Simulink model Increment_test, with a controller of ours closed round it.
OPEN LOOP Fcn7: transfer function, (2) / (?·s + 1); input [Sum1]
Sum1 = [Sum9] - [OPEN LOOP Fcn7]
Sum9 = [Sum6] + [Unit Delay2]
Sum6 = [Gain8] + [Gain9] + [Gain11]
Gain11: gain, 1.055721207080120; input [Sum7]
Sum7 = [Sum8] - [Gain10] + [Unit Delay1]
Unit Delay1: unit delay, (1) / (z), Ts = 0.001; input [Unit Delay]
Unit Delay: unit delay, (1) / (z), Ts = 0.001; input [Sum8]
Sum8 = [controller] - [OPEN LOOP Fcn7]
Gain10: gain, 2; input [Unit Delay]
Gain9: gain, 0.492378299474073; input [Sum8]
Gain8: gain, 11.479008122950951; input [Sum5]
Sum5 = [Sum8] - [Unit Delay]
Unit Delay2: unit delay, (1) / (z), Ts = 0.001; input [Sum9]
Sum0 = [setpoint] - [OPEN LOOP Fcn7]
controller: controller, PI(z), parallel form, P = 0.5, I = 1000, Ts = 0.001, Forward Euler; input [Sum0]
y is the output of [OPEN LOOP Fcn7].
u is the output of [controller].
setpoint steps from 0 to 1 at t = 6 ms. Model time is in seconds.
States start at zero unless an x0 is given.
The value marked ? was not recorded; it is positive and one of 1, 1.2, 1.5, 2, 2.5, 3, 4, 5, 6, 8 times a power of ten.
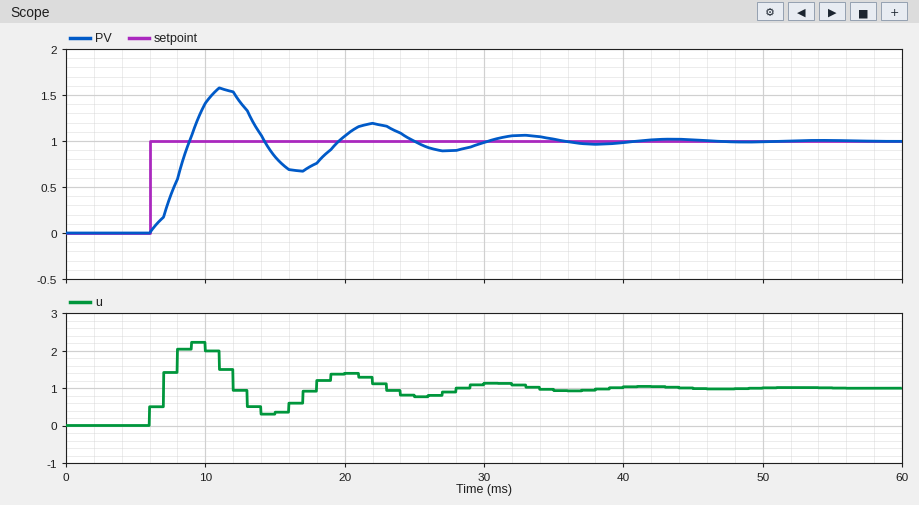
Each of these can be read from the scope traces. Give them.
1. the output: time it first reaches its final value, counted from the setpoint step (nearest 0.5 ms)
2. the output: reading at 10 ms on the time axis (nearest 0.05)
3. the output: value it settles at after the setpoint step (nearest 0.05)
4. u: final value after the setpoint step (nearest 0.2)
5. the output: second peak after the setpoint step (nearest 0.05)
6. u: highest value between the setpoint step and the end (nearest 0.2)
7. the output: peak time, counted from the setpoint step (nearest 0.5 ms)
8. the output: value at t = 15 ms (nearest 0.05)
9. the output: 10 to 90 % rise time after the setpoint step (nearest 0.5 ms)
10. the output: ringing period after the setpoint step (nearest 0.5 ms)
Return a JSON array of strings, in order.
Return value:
["3.0 ms", "1.40", "1.00", "1.0", "1.20", "2.2", "5.0 ms", "0.85", "2.0 ms", "11.0 ms"]
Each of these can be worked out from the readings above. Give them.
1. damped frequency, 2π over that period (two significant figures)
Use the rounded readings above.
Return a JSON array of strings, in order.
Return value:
["0.57 rad/ms"]
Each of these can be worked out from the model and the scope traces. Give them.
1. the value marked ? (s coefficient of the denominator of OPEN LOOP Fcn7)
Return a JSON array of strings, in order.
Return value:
["0.06"]
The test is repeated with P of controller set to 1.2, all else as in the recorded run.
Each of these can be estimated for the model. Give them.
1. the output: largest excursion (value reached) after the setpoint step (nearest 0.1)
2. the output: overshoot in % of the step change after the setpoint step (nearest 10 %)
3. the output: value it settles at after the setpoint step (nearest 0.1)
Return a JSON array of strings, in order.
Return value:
["1.3", "30 %", "1.0"]
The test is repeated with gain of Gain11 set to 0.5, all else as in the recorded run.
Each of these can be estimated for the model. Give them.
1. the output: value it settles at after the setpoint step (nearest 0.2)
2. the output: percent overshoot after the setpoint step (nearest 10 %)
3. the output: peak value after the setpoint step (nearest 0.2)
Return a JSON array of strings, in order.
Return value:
["1.0", "60 %", "1.6"]
